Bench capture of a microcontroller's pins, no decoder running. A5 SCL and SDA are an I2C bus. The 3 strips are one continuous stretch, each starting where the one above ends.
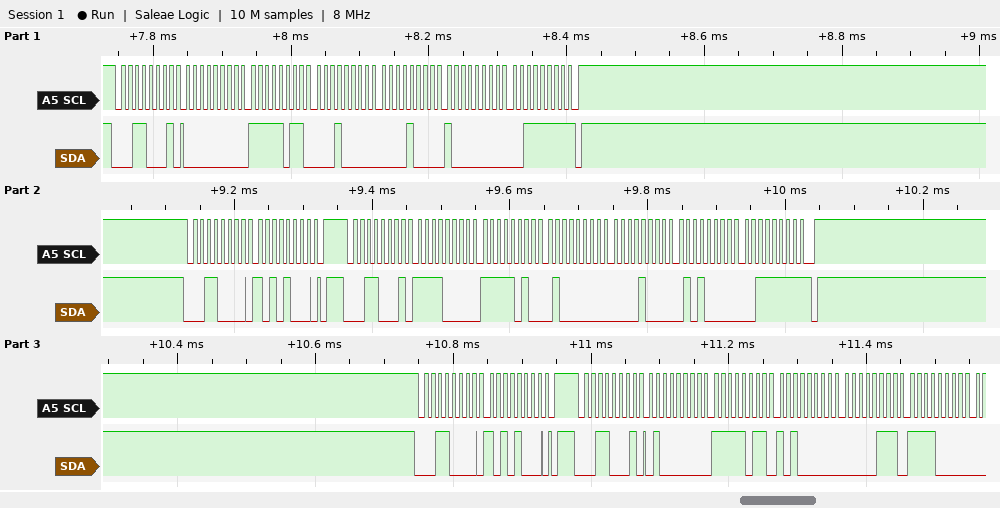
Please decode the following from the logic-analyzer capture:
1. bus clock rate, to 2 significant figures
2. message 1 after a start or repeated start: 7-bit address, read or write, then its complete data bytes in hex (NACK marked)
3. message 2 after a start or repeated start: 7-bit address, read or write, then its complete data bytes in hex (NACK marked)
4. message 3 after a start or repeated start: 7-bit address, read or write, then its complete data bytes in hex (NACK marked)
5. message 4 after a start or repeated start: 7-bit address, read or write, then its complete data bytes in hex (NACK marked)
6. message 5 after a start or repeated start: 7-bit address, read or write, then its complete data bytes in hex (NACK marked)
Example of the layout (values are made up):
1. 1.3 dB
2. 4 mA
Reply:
1. 100 kHz
2. 0x18 read: 00 FB 10 08 80 3F NACK
3. 0x18 write: A8
4. 0x18 read: F0 FA 40 08 50 3F NACK
5. 0x18 write: A8
6. 0x18 read: 40 FB A0 07 F0
